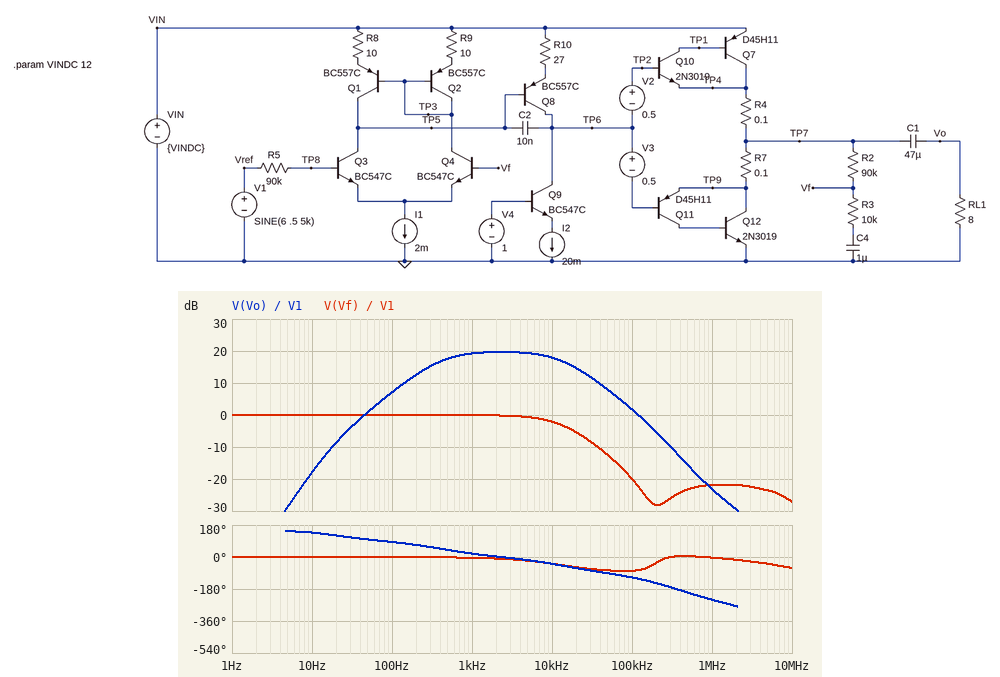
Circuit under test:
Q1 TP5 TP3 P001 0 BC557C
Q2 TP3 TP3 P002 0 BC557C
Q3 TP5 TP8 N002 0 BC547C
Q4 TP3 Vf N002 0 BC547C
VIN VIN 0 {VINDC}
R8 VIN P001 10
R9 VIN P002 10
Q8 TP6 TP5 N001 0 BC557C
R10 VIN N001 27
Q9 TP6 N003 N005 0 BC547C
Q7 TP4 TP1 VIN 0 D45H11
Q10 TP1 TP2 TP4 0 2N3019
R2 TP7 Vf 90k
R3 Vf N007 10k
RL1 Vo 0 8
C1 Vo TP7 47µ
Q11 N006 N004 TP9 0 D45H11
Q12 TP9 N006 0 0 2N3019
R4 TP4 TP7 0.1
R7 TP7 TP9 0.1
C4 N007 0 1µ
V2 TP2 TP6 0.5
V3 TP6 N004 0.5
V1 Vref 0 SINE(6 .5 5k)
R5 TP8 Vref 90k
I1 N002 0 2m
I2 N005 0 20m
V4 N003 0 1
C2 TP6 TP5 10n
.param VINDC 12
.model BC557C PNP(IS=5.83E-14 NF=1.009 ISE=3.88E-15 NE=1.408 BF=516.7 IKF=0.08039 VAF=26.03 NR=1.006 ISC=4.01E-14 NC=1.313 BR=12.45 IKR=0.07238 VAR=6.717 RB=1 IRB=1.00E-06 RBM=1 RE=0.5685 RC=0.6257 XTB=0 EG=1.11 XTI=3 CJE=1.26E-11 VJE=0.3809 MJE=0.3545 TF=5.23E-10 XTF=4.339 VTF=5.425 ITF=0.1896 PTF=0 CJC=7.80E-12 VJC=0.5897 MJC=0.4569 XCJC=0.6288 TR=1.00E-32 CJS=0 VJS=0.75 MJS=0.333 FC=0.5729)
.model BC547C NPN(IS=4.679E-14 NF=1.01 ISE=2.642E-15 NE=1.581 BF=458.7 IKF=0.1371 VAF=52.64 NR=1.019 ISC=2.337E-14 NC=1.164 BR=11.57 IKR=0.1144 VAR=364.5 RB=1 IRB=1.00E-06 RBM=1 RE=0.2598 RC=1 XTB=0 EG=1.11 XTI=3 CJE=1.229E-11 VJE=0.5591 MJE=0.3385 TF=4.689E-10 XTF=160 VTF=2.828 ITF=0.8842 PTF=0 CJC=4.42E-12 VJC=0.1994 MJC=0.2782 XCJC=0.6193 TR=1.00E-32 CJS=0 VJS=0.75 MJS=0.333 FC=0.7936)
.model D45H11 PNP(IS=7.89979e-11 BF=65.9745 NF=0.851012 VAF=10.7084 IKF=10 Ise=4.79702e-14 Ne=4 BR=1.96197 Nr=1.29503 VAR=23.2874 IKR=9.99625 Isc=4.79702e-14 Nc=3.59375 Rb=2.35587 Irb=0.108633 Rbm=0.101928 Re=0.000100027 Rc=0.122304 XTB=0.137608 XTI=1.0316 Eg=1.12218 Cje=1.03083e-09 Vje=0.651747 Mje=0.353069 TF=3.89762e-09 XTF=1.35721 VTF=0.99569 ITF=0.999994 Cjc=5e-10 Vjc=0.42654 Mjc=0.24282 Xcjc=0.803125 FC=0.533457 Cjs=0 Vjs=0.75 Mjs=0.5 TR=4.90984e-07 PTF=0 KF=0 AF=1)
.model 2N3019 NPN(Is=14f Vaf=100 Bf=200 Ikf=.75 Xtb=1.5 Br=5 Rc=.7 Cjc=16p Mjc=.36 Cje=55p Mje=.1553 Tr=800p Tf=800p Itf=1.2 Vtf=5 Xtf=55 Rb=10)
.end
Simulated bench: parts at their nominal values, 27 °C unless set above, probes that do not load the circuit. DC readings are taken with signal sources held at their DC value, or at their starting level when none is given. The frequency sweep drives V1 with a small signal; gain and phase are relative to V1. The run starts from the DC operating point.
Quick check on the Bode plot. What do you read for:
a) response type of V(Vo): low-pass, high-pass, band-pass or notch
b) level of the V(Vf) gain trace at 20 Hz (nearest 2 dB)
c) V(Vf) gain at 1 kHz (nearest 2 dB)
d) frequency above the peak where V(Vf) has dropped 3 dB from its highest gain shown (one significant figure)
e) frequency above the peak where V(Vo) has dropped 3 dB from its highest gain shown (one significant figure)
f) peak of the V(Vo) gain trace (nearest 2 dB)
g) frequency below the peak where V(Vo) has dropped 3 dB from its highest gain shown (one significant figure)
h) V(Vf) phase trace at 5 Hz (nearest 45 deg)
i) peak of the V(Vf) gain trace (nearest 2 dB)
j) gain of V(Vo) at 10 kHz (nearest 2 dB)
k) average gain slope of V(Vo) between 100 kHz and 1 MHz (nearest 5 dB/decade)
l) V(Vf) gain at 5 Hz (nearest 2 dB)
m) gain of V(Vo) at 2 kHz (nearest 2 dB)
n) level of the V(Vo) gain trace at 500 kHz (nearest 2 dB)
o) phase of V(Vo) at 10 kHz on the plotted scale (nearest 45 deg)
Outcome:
band-pass
0 dB
0 dB
10 kHz
10 kHz
20 dB
400 Hz
0 deg
0 dB
18 dB
-25 dB/decade
0 dB
20 dB
-16 dB
-45 deg
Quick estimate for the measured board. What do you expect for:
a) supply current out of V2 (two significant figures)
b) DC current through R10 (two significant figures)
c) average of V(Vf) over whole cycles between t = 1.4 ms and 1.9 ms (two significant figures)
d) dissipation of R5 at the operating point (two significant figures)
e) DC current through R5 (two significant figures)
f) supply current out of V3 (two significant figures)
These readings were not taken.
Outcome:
4.6 µA
20 mA
5.8 V
390 nW
2.1 µA
5.3 µA
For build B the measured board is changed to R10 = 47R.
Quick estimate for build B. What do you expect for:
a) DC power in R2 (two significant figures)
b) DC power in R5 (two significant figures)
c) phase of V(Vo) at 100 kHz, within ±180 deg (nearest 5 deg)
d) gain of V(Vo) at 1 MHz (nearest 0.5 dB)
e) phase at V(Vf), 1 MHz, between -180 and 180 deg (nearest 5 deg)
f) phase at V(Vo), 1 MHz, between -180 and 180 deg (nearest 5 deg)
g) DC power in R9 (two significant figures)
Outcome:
330 nW
400 nW
-125 deg
-19.5 dB
0 deg
105 deg
9.2 µW
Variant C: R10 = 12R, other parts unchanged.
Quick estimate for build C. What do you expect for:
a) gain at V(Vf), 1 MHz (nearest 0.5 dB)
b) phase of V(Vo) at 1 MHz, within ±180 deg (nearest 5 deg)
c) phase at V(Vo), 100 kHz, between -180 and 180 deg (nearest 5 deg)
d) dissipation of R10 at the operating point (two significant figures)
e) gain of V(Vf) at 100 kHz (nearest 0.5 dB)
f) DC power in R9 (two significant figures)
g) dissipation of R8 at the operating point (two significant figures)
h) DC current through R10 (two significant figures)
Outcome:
-21.5 dB
140 deg
-110 deg
4.8 mW
-19.5 dB
9.4 µW
9.6 µW
20 mA
